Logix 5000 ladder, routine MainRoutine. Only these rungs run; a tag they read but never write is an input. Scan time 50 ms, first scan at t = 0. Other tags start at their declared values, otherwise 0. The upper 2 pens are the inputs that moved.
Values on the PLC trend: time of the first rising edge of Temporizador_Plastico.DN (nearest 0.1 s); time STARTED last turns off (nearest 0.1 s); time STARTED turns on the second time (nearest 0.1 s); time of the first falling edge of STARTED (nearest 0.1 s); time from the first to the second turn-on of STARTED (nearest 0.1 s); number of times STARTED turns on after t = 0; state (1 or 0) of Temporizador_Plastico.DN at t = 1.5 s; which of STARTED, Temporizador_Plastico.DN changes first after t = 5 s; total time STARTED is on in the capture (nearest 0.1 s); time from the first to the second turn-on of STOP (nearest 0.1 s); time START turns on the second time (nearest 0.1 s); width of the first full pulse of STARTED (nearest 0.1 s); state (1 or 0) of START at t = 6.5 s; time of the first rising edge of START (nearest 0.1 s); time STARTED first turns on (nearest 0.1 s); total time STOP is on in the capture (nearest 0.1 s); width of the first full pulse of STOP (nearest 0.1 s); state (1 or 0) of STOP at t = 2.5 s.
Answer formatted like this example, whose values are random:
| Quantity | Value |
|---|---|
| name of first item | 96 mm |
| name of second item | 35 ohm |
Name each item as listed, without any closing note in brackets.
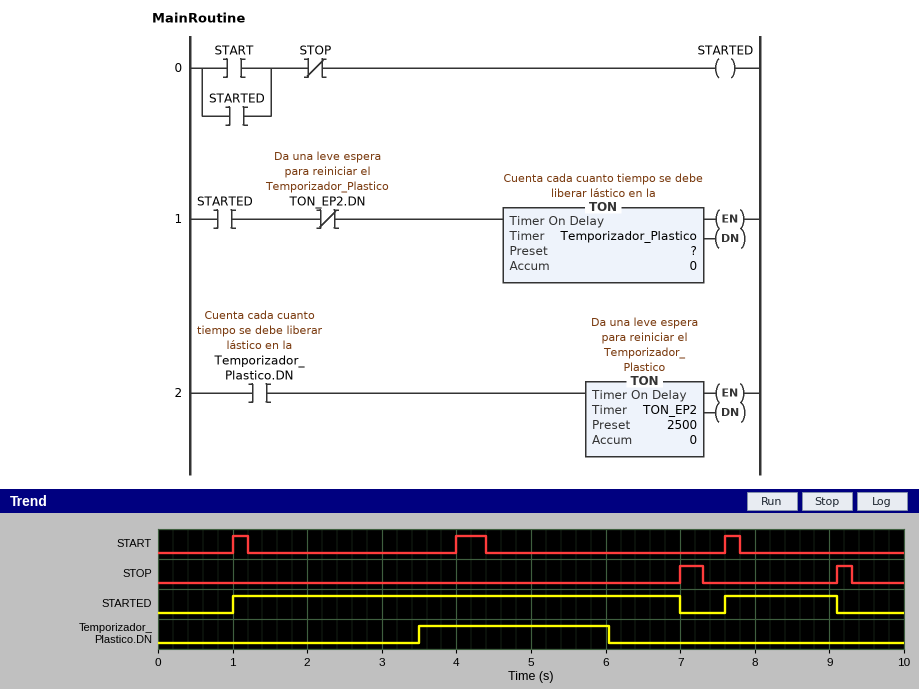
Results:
| Quantity | Value |
|---|---|
| time of the first rising edge of Temporizador_Plastico.DN | 3.5 s |
| time STARTED last turns off | 9.1 s |
| time STARTED turns on the second time | 7.6 s |
| time of the first falling edge of STARTED | 7.0 s |
| time from the first to the second turn-on of STARTED | 6.6 s |
| number of times STARTED turns on after t = 0 | 2 |
| state (1 or 0) of Temporizador_Plastico.DN at t = 1.5 s | 0 |
| which of STARTED, Temporizador_Plastico.DN changes first after t = 5 s | Temporizador_Plastico.DN |
| total time STARTED is on in the capture | 7.5 s |
| time from the first to the second turn-on of STOP | 2.1 s |
| time START turns on the second time | 4.0 s |
| width of the first full pulse of STARTED | 6.0 s |
| state (1 or 0) of START at t = 6.5 s | 0 |
| time of the first rising edge of START | 1.0 s |
| time STARTED first turns on | 1.0 s |
| total time STOP is on in the capture | 0.5 s |
| width of the first full pulse of STOP | 0.3 s |
| state (1 or 0) of STOP at t = 2.5 s | 0 |
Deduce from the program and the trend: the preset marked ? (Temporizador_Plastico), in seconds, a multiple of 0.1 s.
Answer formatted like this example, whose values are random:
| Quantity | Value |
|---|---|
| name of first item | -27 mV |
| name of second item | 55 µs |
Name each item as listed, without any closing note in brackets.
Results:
| Quantity | Value |
|---|---|
| the preset marked ? (Temporizador_Plastico), in seconds, a multiple of 0.1 s | 2.5 s |
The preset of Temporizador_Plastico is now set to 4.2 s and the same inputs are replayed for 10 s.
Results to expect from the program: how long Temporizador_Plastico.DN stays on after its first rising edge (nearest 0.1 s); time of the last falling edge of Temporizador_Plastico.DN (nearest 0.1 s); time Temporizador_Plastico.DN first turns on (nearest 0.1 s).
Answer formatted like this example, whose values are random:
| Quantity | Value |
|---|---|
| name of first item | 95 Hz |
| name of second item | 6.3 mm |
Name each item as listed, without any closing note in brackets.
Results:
| Quantity | Value |
|---|---|
| how long Temporizador_Plastico.DN stays on after its first rising edge | 1.8 s |
| time of the last falling edge of Temporizador_Plastico.DN | 7.0 s |
| time Temporizador_Plastico.DN first turns on | 5.2 s |
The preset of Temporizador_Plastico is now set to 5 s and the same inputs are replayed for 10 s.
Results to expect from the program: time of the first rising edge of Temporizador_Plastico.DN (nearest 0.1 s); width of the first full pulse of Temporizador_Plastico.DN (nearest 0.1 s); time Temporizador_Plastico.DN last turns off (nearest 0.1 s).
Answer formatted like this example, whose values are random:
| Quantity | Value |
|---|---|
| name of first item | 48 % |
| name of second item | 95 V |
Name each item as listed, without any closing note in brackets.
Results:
| Quantity | Value |
|---|---|
| time of the first rising edge of Temporizador_Plastico.DN | 6.0 s |
| width of the first full pulse of Temporizador_Plastico.DN | 1.0 s |
| time Temporizador_Plastico.DN last turns off | 7.0 s |
